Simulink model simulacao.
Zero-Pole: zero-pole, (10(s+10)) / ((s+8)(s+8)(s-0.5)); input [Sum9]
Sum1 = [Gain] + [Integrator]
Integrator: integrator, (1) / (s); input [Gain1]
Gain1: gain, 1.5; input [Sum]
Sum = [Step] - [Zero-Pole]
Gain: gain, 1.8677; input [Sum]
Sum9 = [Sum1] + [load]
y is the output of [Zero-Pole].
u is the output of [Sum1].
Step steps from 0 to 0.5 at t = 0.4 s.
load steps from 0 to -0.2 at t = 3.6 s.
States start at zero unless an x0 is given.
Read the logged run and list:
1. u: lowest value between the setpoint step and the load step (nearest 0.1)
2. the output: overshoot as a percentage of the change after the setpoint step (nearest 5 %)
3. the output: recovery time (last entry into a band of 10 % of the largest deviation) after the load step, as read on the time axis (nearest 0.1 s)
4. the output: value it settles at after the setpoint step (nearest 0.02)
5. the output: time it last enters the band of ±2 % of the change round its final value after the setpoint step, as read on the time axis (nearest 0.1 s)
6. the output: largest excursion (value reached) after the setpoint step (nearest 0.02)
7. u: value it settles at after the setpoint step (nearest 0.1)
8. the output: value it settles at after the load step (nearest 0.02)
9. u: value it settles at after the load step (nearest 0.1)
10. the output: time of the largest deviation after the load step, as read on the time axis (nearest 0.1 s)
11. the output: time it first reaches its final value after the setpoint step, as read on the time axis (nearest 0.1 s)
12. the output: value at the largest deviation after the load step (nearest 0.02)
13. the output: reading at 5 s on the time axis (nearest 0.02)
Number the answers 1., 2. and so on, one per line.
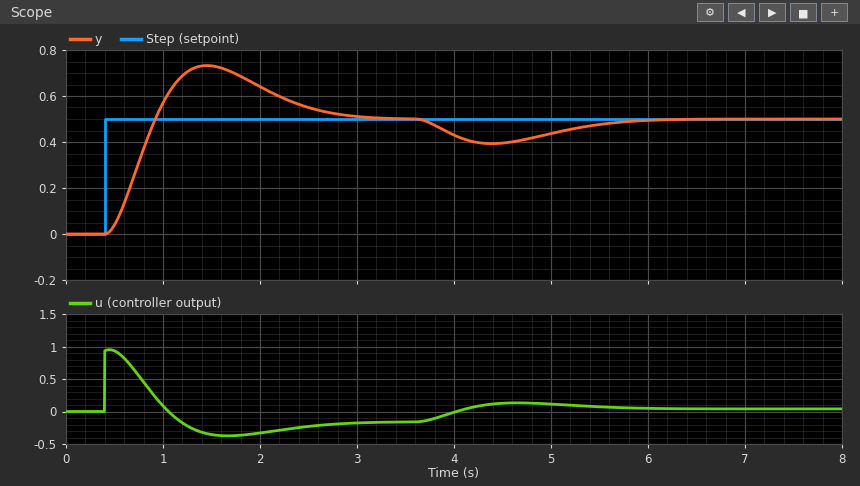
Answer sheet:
1. -0.4
2. 45 %
3. 5.8 s
4. 0.50
5. 3.0 s
6. 0.74
7. -0.2
8. 0.50
9. 0.0
10. 4.4 s
11. 0.9 s
12. 0.40
13. 0.44
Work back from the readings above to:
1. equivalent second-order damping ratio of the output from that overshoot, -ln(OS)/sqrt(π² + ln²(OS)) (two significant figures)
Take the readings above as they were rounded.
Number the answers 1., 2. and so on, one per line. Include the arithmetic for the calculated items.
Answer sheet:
1. ln(0.45) = -0.799; 0.799 / sqrt(9.870 + 0.638) = 0.25
